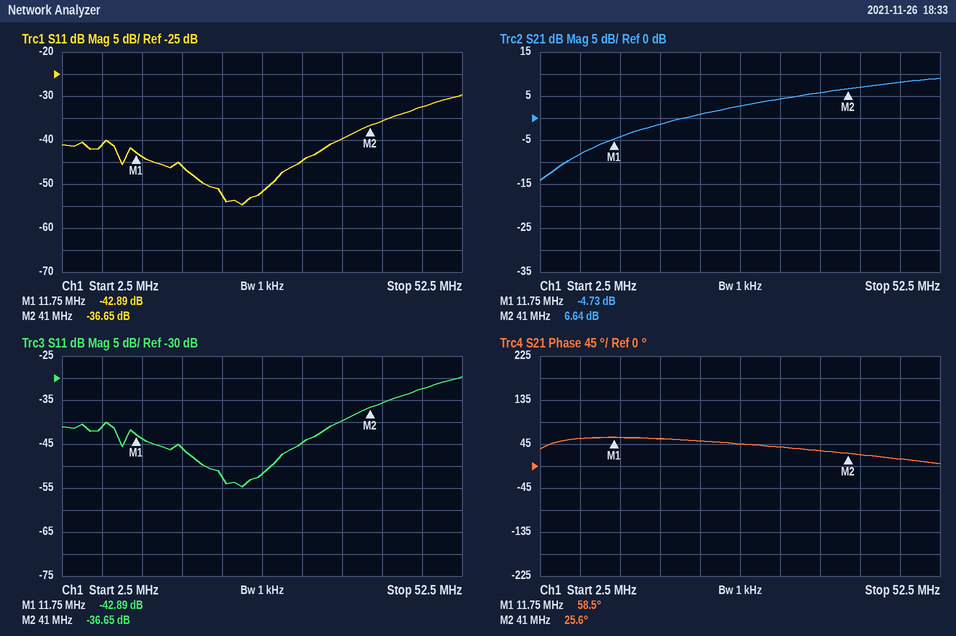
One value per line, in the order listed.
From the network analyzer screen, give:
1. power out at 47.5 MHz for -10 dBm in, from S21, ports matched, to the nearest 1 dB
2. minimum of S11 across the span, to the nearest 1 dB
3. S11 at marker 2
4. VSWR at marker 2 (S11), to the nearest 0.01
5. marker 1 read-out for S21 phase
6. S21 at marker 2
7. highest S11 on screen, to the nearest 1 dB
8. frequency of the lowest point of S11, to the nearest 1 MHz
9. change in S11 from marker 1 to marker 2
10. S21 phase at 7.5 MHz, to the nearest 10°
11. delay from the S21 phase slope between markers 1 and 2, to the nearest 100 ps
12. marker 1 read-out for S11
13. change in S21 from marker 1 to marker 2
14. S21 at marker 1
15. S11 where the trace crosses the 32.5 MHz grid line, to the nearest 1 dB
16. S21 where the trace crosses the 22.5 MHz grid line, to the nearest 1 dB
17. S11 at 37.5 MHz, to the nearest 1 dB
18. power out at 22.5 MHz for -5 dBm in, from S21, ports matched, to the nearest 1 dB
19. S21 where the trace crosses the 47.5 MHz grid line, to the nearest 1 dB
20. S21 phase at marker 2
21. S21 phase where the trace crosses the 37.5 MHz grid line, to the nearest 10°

-2 dBm
-55 dB
-36.65 dB
1.03
58.5°
6.64 dB
-30 dB
25 MHz
6.24 dB
60°
3.1 ns
-42.89 dB
11.37 dB
-4.73 dB
-45 dB
1 dB
-40 dB
-4 dBm
8 dB
25.6°
30°
